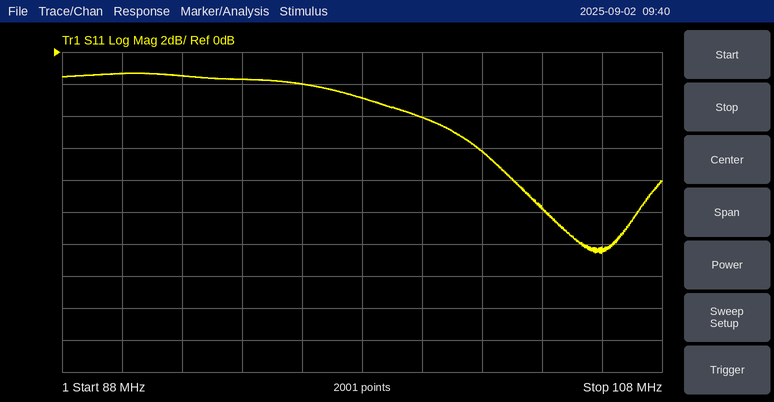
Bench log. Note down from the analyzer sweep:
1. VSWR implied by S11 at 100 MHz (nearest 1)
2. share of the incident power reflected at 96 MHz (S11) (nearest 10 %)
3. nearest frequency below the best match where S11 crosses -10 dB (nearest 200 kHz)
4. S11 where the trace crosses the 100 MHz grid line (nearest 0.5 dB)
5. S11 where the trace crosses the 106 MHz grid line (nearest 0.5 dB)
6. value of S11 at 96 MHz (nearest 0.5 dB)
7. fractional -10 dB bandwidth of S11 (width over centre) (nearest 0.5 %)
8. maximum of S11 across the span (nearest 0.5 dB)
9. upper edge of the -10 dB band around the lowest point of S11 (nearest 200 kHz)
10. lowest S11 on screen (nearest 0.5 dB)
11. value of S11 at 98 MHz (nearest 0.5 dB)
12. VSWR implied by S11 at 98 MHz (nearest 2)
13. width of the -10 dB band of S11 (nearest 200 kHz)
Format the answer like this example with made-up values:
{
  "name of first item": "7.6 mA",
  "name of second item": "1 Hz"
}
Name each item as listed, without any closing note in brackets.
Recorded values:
{
  "VSWR implied by S11 at 100 MHz": "4",
  "share of the incident power reflected at 96 MHz (S11)": "60 %",
  "nearest frequency below the best match where S11 crosses -10 dB": "104.2 MHz",
  "S11 where the trace crosses the 100 MHz grid line": "-4.0 dB",
  "S11 where the trace crosses the 106 MHz grid line": "-12.5 dB",
  "value of S11 at 96 MHz": "-2.0 dB",
  "fractional -10 dB bandwidth of S11 (width over centre)": "3.0 %",
  "maximum of S11 across the span": "-1.5 dB",
  "upper edge of the -10 dB band around the lowest point of S11": "107.2 MHz",
  "lowest S11 on screen": "-12.5 dB",
  "value of S11 at 98 MHz": "-3.0 dB",
  "VSWR implied by S11 at 98 MHz": "6",
  "width of the -10 dB band of S11": "3.0 MHz"
}
